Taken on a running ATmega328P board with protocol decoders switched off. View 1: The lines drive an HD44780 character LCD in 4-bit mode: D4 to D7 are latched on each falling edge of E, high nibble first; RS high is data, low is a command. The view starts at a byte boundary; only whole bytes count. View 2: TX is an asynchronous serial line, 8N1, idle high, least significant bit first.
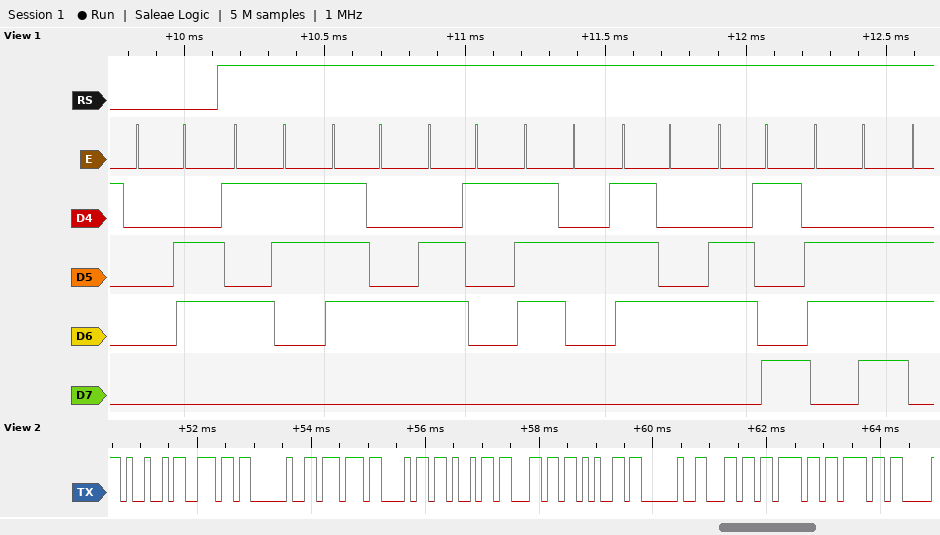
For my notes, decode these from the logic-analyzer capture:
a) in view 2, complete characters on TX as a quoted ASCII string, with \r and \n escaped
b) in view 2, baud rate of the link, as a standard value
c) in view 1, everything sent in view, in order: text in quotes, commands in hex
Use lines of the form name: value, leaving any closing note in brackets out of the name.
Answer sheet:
in view 2, complete characters on TX as a quoted ASCII string, with \r and \n escaped: "In while loo"
in view 2, baud rate of the link, as a standard value: 9600 baud
in view 1, everything sent in view, in order: text in quotes, commands in hex: 0x06 "Startin"
